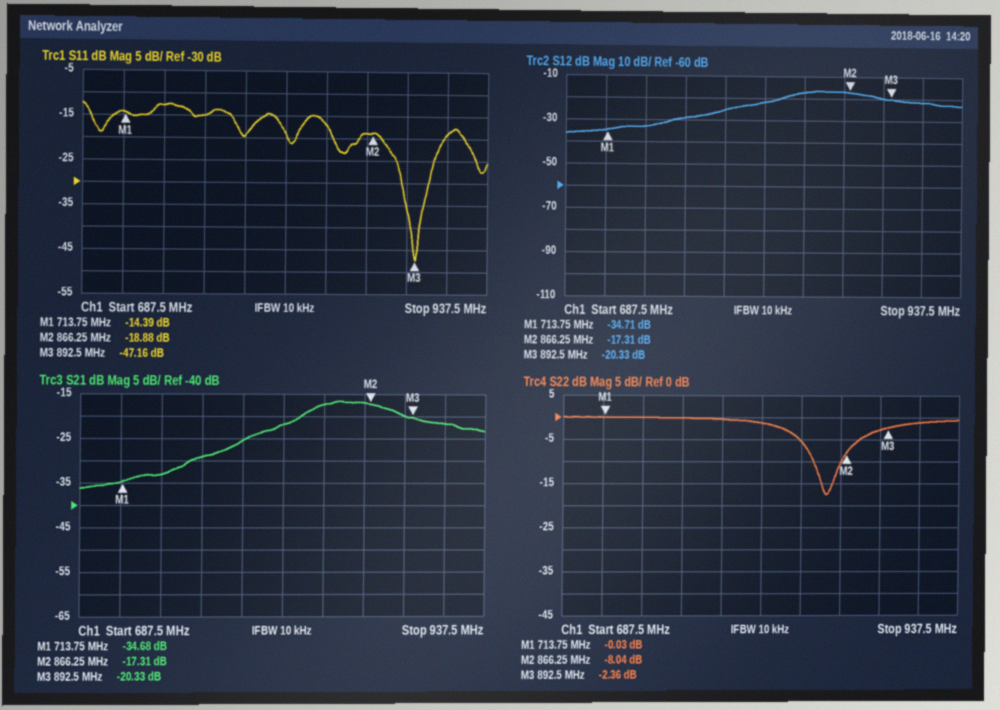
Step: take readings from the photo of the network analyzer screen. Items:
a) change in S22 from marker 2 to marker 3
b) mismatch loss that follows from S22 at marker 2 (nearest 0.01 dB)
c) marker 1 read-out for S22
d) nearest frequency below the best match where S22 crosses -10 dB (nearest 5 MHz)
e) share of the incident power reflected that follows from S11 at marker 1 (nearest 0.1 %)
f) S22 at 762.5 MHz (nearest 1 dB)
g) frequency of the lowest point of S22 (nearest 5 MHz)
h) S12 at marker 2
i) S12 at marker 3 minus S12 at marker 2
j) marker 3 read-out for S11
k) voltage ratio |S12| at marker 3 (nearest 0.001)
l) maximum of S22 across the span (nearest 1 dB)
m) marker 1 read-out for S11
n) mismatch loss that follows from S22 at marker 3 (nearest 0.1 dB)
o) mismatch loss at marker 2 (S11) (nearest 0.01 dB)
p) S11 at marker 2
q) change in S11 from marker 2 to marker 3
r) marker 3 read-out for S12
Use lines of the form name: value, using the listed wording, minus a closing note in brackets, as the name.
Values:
change in S22 from marker 2 to marker 3: 5.68 dB
mismatch loss that follows from S22 at marker 2: 0.74 dB
marker 1 read-out for S22: -0.03 dB
nearest frequency below the best match where S22 crosses -10 dB: 845 MHz
share of the incident power reflected that follows from S11 at marker 1: 3.6 %
S22 at 762.5 MHz: 0 dB
frequency of the lowest point of S22: 855 MHz
S12 at marker 2: -17.31 dB
S12 at marker 3 minus S12 at marker 2: -3.02 dB
marker 3 read-out for S11: -47.16 dB
voltage ratio |S12| at marker 3: 0.096
maximum of S22 across the span: 0 dB
marker 1 read-out for S11: -14.39 dB
mismatch loss that follows from S22 at marker 3: 3.8 dB
mismatch loss at marker 2 (S11): 0.06 dB
S11 at marker 2: -18.88 dB
change in S11 from marker 2 to marker 3: -28.28 dB
marker 3 read-out for S12: -20.33 dB
